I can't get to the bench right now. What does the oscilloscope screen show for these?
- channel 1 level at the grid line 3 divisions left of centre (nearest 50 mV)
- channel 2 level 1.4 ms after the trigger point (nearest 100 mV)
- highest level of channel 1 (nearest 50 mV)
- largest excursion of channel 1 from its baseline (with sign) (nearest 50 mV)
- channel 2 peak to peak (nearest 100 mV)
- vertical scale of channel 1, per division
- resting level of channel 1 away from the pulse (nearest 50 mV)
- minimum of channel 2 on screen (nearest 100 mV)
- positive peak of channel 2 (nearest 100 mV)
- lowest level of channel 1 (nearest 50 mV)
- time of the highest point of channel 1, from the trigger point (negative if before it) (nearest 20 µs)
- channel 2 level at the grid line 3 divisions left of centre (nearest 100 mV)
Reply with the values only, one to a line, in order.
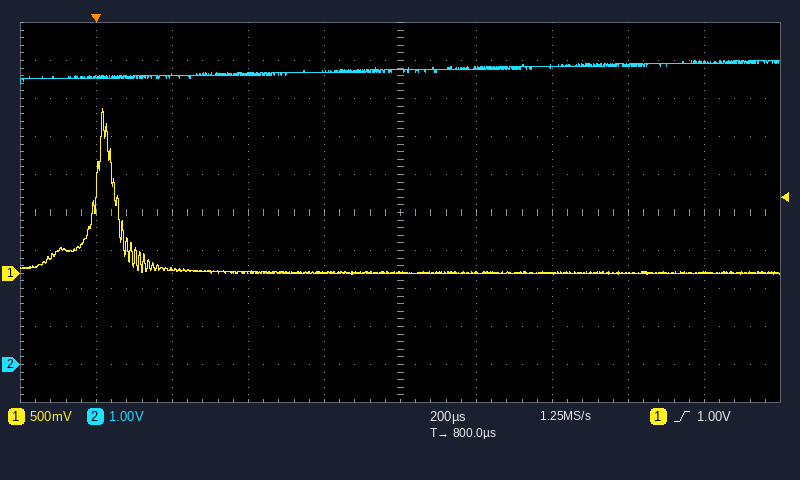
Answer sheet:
50 mV
7.9 V
2.15 V
+2.15 V
600 mV
500 mV
0 mV
7.4 V
8.0 V
0 mV
+20 µs
7.6 V
